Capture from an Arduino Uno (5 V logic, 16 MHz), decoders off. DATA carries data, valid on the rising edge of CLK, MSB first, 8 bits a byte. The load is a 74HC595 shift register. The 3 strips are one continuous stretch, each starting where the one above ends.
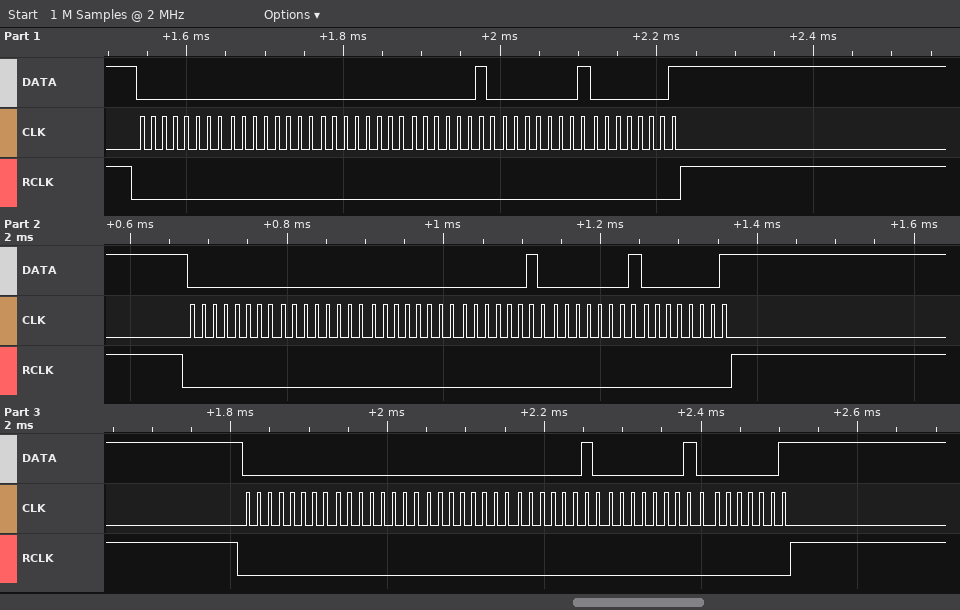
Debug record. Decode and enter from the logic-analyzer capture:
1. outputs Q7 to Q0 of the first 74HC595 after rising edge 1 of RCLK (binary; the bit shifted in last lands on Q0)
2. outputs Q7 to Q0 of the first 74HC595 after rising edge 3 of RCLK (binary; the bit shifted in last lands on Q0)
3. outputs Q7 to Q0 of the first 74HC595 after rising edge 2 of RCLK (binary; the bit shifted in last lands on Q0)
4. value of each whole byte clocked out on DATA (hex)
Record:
00000001
00000001
00000001
00 00 00 02 01 01 00 00 00 02 01 01 00 00 00 02 01 01
